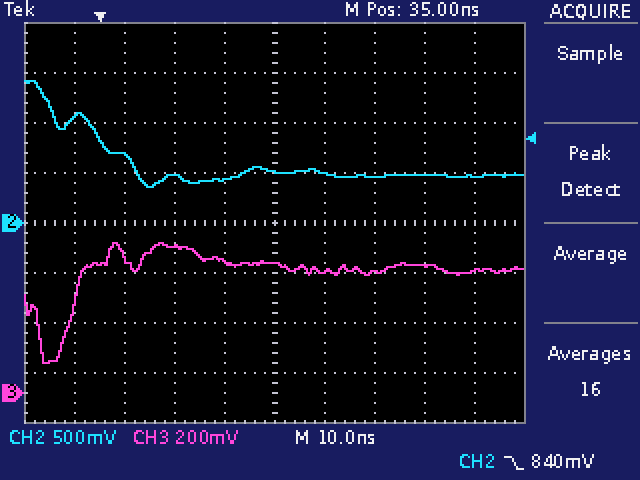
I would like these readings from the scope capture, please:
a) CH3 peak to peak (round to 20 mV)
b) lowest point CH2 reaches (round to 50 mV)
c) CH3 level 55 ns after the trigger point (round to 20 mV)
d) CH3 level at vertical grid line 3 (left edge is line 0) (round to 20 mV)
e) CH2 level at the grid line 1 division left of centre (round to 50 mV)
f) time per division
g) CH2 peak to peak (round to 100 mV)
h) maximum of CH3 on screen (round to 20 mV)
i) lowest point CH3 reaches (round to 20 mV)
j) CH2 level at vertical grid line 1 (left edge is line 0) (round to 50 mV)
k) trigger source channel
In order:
480 mV
350 mV
480 mV
580 mV
450 mV
10 ns
1.10 V
600 mV
120 mV
1.05 V
CH2
